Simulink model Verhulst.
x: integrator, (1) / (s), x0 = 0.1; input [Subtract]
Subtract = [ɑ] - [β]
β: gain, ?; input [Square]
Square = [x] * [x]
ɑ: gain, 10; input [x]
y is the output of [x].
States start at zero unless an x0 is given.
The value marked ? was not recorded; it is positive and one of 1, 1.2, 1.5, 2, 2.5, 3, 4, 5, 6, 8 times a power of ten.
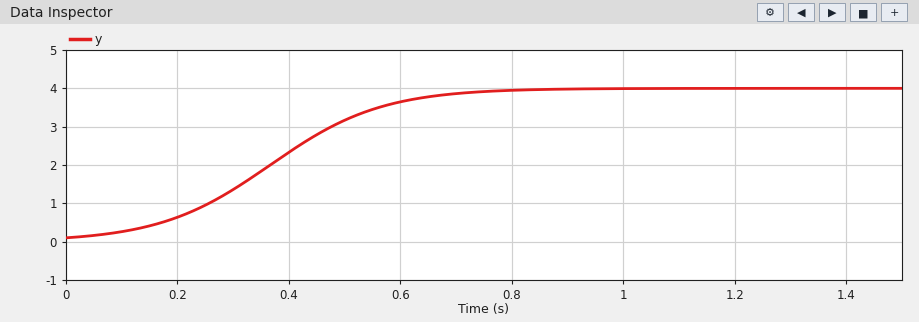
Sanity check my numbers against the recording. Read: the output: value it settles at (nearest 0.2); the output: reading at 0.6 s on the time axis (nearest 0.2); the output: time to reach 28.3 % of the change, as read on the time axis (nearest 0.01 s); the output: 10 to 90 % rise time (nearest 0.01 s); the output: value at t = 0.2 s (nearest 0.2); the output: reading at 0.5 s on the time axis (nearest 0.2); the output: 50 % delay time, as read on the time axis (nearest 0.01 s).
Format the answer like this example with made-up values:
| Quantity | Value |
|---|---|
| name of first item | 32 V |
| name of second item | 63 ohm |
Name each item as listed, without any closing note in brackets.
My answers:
| Quantity | Value |
|---|---|
| the output: value it settles at | 4.0 |
| the output: reading at 0.6 s on the time axis | 3.6 |
| the output: time to reach 28.3 % of the change, as read on the time axis | 0.28 s |
| the output: 10 to 90 % rise time | 0.42 s |
| the output: value at t = 0.2 s | 0.6 |
| the output: reading at 0.5 s on the time axis | 3.2 |
| the output: 50 % delay time, as read on the time axis | 0.37 s |
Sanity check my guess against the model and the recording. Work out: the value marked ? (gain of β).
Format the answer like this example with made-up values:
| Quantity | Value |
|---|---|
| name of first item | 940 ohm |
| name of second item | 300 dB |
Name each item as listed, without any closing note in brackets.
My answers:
| Quantity | Value |
|---|---|
| the value marked ? | 2.5 |
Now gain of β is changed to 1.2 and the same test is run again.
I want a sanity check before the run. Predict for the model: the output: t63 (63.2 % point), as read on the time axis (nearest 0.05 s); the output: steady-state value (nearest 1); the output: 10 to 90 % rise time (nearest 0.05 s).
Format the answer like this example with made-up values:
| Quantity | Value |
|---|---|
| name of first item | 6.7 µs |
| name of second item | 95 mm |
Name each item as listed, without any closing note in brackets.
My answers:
| Quantity | Value |
|---|---|
| the output: t63 (63.2 % point), as read on the time axis | 0.50 s |
| the output: steady-state value | 8 |
| the output: 10 to 90 % rise time | 0.45 s |
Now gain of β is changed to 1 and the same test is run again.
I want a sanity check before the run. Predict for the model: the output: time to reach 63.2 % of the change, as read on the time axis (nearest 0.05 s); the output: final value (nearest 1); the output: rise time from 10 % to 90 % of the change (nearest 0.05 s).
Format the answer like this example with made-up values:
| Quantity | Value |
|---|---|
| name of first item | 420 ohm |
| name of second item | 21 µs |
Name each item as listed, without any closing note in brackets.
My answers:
| Quantity | Value |
|---|---|
| the output: time to reach 63.2 % of the change, as read on the time axis | 0.50 s |
| the output: final value | 10 |
| the output: rise time from 10 % to 90 % of the change | 0.45 s |
